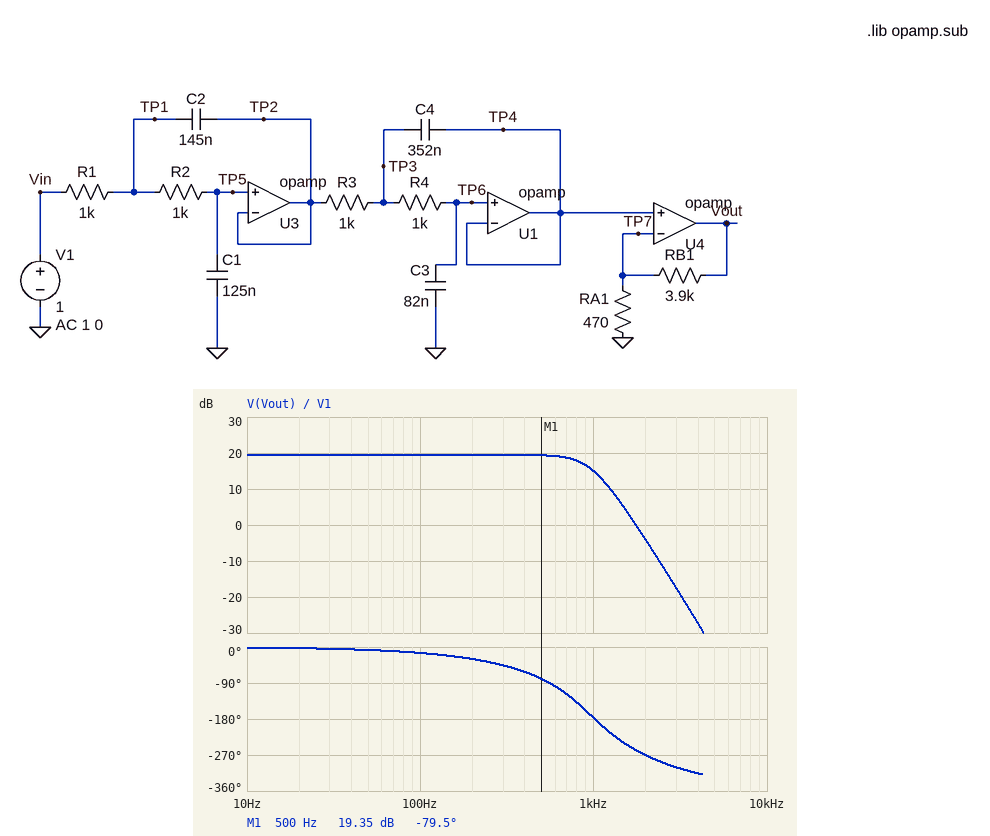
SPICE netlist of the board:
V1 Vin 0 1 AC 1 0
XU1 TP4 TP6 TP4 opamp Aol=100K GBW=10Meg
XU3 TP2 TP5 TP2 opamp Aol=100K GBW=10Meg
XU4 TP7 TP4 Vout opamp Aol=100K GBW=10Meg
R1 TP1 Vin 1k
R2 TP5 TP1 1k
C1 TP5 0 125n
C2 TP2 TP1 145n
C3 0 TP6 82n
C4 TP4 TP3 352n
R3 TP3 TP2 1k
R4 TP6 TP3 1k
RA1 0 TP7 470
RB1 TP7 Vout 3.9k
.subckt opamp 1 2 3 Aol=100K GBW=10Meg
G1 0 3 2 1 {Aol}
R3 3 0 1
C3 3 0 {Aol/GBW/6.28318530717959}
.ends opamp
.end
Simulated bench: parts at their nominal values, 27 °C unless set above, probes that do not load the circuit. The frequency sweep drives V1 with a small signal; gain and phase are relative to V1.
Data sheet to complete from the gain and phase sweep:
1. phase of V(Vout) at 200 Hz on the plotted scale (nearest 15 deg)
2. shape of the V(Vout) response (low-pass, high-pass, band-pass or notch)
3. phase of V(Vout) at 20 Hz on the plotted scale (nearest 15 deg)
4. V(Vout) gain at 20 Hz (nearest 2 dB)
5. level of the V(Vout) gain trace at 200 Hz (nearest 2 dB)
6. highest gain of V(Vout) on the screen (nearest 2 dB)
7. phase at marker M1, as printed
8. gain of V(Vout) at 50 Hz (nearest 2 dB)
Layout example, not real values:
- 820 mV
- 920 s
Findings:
- -30 deg
- low-pass
- 0 deg
- 20 dB
- 20 dB
- 20 dB
- -79.5 deg
- 20 dB
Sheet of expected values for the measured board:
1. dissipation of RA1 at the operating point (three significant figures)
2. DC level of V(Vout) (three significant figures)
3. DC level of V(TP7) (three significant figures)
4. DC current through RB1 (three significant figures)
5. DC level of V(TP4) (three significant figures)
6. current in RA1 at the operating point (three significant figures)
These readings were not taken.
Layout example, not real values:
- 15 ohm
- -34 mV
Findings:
- 2.13 mW
- 9.30 V
- 1.00 V
- 2.13 mA
- 1.00 V
- 2.13 mA
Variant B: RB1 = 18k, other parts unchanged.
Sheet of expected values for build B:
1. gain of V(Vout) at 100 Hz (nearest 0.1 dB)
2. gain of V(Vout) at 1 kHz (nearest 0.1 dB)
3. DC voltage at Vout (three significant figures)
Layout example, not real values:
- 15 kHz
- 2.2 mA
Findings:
- 31.9 dB
- 27.5 dB
- 39.3 V
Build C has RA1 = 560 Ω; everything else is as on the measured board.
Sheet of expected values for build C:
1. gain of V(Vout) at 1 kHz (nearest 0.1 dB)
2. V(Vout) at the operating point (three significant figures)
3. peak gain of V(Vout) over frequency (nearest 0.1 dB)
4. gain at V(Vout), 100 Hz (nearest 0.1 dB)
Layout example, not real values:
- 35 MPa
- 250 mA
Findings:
- 13.6 dB
- 7.96 V
- 18.1 dB
- 18.0 dB
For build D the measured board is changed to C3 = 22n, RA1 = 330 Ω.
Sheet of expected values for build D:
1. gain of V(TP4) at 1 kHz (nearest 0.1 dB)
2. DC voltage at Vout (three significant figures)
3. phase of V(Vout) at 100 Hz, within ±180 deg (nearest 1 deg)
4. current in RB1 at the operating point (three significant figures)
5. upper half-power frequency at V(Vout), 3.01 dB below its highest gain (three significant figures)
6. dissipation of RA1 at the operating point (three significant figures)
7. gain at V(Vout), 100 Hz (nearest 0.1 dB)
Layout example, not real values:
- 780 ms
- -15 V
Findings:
- -1.5 dB
- 12.8 V
- -11 deg
- 3.03 mA
- 1.72 kHz
- 3.03 mW
- 22.1 dB
